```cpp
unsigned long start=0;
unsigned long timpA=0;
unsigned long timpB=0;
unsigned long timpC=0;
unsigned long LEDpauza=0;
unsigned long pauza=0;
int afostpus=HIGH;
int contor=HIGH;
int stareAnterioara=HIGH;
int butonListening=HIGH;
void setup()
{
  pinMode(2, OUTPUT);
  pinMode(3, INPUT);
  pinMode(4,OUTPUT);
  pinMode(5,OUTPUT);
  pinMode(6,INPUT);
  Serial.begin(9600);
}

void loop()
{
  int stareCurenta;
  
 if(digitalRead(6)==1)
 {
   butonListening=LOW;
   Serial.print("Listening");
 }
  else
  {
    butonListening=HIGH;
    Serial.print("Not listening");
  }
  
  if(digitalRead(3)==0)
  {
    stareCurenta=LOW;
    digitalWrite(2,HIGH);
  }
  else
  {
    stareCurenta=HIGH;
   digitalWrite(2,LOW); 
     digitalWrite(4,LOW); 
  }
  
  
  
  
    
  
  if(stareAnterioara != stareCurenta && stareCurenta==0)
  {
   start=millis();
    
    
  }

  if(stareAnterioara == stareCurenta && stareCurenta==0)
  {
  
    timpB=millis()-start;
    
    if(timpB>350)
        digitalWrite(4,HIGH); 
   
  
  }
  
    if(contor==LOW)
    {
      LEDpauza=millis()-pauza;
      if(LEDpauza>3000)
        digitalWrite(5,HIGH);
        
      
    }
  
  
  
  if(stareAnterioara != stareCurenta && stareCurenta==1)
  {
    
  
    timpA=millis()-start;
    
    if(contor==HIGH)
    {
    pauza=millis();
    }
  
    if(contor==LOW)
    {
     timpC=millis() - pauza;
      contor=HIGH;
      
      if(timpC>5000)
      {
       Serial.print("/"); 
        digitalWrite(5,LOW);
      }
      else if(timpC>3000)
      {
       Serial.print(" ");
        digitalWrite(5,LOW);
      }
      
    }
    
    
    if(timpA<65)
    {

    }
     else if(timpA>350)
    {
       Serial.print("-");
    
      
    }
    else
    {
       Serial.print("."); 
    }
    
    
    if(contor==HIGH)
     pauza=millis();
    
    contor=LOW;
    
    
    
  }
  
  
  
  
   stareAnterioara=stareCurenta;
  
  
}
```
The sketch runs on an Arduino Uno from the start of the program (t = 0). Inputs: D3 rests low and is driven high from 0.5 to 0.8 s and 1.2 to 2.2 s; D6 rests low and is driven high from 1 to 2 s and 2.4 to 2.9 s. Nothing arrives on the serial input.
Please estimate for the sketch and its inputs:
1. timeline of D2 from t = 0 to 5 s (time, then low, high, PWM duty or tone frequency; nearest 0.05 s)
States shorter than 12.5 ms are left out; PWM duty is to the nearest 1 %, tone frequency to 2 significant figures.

0 s high; 0.5 s low; 0.8 s high; 1.2 s low; 2.2 s high
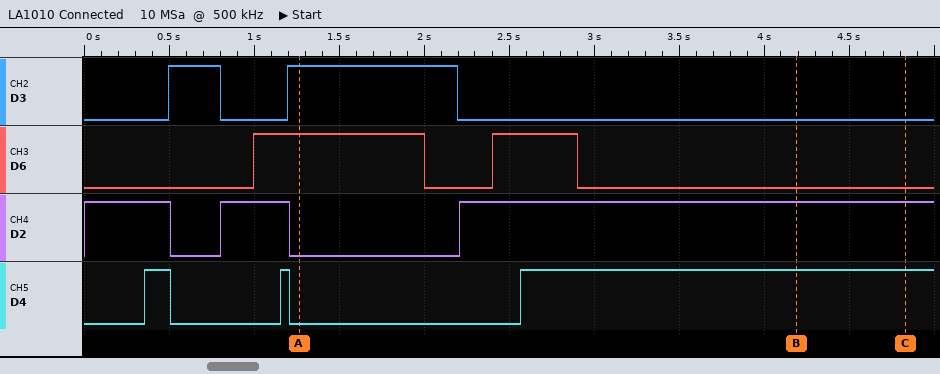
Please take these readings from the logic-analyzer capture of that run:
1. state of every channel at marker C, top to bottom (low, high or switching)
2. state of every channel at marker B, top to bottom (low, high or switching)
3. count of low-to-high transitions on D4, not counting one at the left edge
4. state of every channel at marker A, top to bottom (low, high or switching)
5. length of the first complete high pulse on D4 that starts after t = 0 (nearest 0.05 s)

D3 low, D6 low, D2 high, D4 high
D3 low, D6 low, D2 high, D4 high
3
D3 high, D6 high, D2 low, D4 low
0.15 s
